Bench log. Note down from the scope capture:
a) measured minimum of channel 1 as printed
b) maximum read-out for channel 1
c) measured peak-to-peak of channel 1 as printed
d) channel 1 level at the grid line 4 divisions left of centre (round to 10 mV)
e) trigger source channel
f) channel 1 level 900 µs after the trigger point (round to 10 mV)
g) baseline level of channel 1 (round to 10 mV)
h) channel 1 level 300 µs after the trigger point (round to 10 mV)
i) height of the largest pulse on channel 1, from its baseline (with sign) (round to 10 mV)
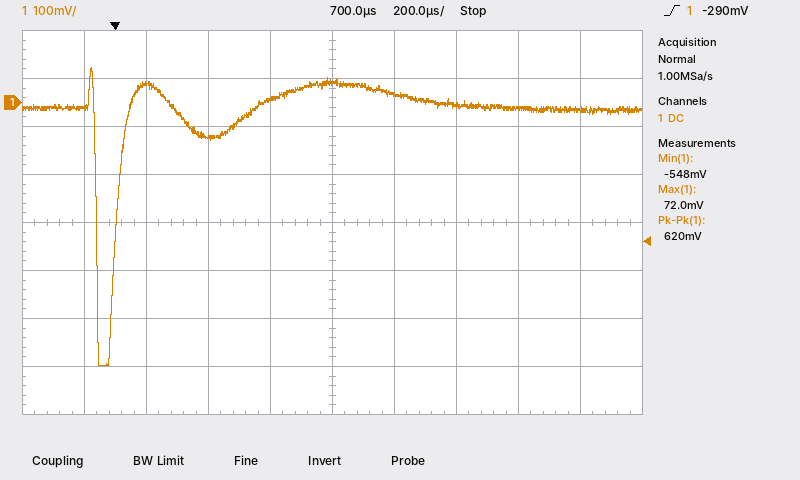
-548 mV
72.0 mV
620 mV
-10 mV
channel 1
20 mV
-10 mV
-70 mV
-540 mV
